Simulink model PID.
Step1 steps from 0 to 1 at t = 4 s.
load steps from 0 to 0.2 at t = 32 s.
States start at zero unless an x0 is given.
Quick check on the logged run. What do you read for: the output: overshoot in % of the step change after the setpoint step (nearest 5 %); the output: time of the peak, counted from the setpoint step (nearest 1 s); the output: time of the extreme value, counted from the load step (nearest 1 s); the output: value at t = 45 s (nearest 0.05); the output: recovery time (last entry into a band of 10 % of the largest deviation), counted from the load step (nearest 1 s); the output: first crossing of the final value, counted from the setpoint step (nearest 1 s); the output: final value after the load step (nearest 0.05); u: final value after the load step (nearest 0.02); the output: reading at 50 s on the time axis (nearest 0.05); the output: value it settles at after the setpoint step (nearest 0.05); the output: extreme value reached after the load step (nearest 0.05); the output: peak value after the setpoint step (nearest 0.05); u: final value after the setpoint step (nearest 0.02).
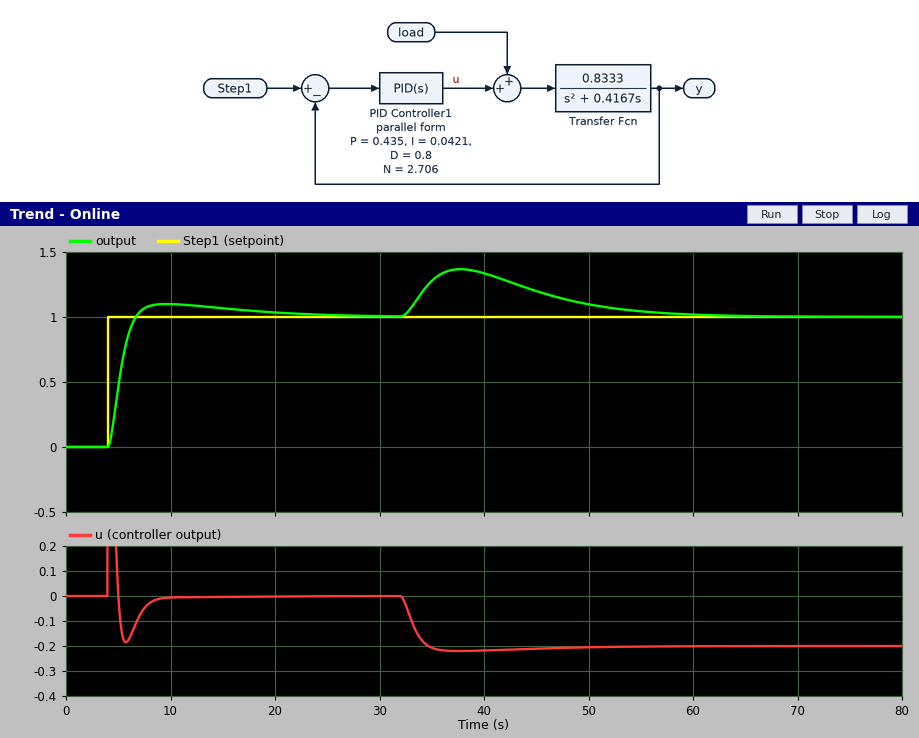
10 %
6 s
6 s
1.20
24 s
3 s
1.00
-0.20
1.10
1.00
1.35
1.10
0.00
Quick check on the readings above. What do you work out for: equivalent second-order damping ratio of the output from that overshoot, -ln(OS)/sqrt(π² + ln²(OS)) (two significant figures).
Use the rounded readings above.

0.59
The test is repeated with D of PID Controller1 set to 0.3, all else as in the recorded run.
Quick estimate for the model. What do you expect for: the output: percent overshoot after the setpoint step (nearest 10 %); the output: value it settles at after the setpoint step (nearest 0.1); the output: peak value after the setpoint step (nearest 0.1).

30 %
1.0
1.3
